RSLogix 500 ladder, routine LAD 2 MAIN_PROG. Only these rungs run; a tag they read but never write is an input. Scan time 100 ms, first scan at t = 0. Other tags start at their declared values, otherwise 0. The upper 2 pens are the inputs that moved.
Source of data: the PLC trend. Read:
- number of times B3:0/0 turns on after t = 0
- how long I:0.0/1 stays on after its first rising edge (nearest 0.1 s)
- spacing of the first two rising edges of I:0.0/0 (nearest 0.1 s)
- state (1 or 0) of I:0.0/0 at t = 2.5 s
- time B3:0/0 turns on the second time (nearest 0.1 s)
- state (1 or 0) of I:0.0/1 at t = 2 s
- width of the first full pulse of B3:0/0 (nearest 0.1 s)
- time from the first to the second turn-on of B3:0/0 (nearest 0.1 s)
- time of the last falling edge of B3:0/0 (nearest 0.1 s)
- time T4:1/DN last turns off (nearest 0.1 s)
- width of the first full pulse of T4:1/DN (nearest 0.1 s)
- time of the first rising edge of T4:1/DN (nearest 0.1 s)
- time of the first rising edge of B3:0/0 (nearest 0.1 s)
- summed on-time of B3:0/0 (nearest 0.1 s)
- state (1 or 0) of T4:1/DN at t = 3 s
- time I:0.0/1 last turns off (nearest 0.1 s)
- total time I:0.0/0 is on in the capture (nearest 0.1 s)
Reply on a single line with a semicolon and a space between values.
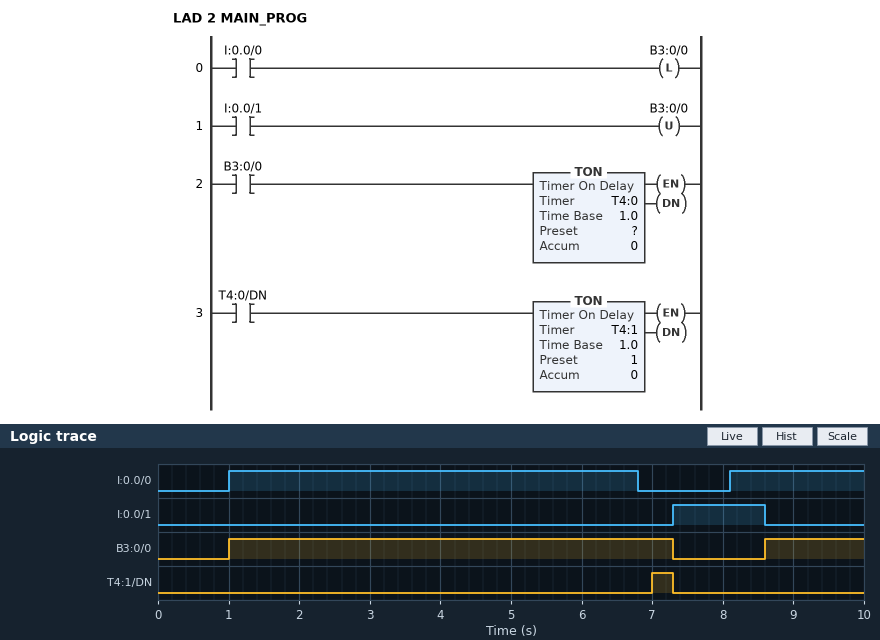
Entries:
2; 1.3 s; 7.1 s; 1; 8.6 s; 0; 6.3 s; 7.6 s; 7.3 s; 7.3 s; 0.3 s; 7.0 s; 1.0 s; 7.7 s; 0; 8.6 s; 7.7 s
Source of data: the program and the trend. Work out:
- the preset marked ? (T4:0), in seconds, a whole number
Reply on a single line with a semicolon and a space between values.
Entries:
5 s
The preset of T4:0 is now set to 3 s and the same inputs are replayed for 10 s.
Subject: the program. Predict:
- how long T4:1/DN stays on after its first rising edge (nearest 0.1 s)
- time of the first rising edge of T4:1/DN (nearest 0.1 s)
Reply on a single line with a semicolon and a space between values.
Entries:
2.3 s; 5.0 s
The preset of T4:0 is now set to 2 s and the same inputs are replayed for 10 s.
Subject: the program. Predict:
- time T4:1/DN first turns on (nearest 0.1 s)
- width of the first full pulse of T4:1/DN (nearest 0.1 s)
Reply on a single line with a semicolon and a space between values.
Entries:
4.0 s; 3.3 s
